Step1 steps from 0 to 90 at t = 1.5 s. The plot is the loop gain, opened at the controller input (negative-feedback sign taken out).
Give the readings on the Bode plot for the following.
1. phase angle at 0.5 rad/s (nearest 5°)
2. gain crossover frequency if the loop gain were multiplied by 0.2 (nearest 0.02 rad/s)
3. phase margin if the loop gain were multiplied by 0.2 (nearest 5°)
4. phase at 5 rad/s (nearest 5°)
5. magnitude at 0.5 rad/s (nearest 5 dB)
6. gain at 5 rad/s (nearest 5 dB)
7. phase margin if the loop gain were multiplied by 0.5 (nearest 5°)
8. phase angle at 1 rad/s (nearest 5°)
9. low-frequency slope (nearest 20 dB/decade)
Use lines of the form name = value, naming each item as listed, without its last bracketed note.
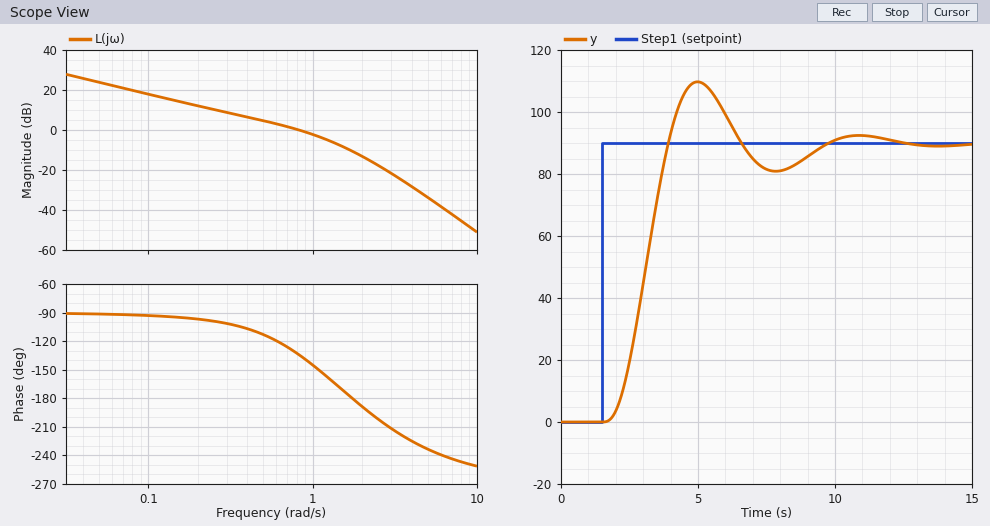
phase angle at 0.5 rad/s = -115°
gain crossover frequency if the loop gain were multiplied by 0.2 = 0.16 rad/s
phase margin if the loop gain were multiplied by 0.2 = 85°
phase at 5 rad/s = -235°
magnitude at 0.5 rad/s = 5 dB
gain at 5 rad/s = -35 dB
phase margin if the loop gain were multiplied by 0.5 = 70°
phase angle at 1 rad/s = -145°
low-frequency slope = -20 dB/decade
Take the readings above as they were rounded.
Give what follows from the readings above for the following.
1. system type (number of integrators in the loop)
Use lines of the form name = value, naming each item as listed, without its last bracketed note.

system type = 1
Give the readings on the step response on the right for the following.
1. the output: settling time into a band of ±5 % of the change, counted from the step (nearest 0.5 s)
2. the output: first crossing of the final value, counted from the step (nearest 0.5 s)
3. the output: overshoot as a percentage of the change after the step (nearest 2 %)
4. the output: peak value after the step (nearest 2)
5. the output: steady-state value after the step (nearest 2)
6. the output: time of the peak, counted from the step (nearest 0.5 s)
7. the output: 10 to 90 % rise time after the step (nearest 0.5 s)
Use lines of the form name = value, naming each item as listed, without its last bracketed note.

the output: settling time into a band of ±5 % of the change, counted from the step = 7.5 s
the output: first crossing of the final value, counted from the step = 2.5 s
the output: overshoot as a percentage of the change after the step = 22 %
the output: peak value after the step = 110
the output: steady-state value after the step = 90
the output: time of the peak, counted from the step = 3.5 s
the output: 10 to 90 % rise time after the step = 1.5 s
